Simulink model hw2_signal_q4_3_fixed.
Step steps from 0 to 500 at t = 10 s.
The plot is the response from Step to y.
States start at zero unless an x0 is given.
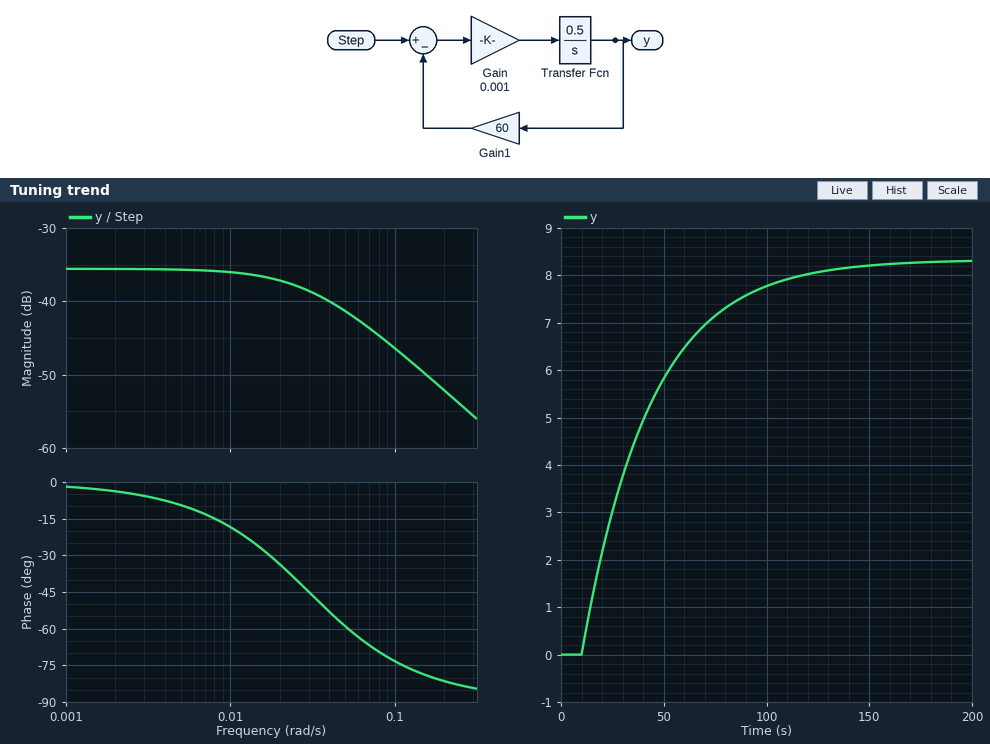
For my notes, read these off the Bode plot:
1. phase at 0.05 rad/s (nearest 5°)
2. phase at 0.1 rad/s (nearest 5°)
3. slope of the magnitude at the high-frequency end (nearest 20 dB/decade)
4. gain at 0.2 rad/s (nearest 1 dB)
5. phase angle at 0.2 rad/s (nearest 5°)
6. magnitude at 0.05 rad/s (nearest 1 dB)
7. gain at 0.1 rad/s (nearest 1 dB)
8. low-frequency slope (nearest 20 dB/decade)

-60°
-75°
-20 dB/decade
-52 dB
-80°
-41 dB
-46 dB
0 dB/decade
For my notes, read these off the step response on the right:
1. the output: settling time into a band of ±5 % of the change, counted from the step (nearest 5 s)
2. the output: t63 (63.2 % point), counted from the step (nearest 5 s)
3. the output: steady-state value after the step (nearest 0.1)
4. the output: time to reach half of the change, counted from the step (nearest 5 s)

100 s
35 s
8.3
25 s
